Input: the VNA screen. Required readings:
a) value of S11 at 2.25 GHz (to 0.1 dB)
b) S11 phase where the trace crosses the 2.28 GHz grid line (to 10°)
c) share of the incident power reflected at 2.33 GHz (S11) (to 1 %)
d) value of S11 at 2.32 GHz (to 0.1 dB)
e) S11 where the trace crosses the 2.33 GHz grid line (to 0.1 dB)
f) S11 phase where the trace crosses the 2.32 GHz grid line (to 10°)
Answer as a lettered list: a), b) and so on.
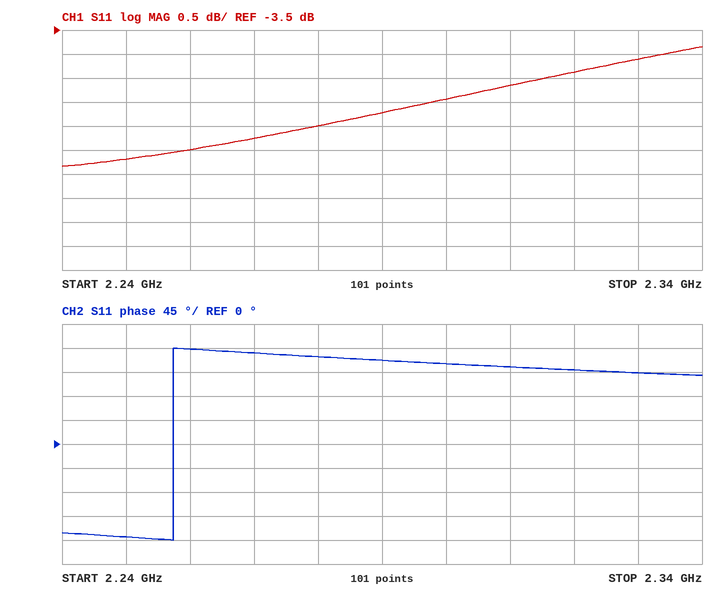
a) -6.2 dB
b) 160°
c) 39 %
d) -4.4 dB
e) -4.1 dB
f) 140°
